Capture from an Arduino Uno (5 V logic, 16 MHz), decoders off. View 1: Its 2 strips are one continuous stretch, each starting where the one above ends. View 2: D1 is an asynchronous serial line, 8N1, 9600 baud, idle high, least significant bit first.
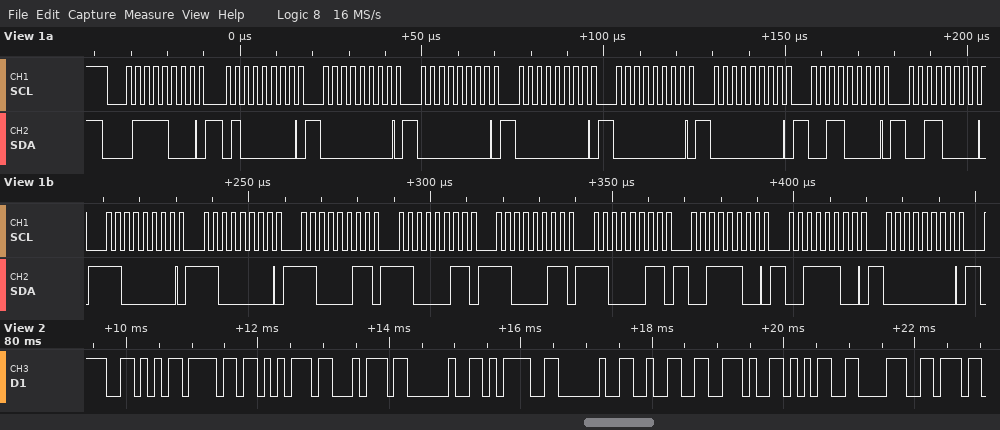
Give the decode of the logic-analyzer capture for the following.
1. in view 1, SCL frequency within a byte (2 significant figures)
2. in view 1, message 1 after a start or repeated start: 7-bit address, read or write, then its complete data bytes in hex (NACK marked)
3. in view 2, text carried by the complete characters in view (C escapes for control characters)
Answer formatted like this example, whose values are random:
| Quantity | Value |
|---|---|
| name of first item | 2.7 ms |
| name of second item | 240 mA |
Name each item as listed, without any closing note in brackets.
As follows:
| Quantity | Value |
|---|---|
| in view 1, SCL frequency within a byte | 400 kHz |
| in view 1, message 1 after a start or repeated start: 7-bit address, read or write, then its complete data bytes in hex | 0x3C write: 40 00 00 00 00 00 30 30 C0 C0 C3 C3 C3 C3 3C 3C 00 |
| in view 2, text carried by the complete characters in view | "Vout = 2.58" |
